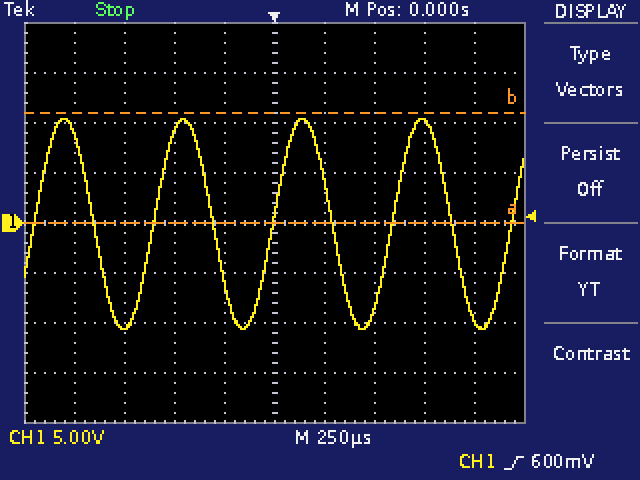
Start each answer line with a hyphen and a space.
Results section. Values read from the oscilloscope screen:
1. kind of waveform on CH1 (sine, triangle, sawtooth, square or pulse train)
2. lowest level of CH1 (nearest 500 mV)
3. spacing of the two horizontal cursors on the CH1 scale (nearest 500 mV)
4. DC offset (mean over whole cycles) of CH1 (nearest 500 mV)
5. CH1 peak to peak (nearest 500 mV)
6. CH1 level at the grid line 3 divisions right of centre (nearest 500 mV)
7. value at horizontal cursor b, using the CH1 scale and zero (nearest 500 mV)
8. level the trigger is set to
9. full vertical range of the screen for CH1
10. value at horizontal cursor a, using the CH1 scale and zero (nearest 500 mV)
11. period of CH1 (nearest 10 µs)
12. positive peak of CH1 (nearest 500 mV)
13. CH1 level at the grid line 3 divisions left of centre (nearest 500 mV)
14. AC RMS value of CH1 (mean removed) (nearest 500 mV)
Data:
- sine
- -10.5 V
- 11.0 V
- 0.0 V
- 21.0 V
- 10.0 V
- 11.0 V
- 600 mV
- 40 V
- 0.0 V
- 600 µs
- 10.5 V
- -10.5 V
- 7.5 V
